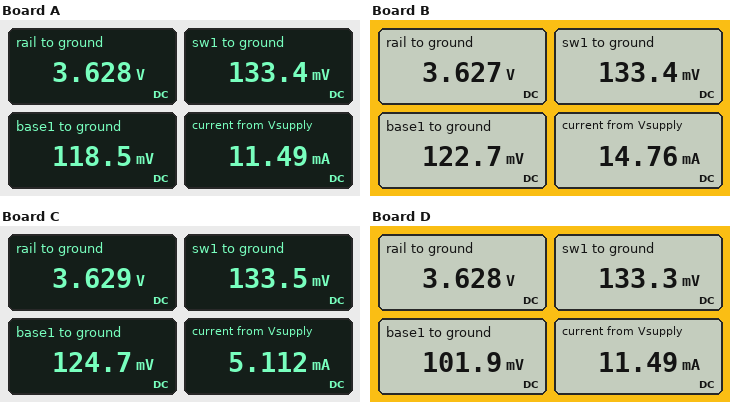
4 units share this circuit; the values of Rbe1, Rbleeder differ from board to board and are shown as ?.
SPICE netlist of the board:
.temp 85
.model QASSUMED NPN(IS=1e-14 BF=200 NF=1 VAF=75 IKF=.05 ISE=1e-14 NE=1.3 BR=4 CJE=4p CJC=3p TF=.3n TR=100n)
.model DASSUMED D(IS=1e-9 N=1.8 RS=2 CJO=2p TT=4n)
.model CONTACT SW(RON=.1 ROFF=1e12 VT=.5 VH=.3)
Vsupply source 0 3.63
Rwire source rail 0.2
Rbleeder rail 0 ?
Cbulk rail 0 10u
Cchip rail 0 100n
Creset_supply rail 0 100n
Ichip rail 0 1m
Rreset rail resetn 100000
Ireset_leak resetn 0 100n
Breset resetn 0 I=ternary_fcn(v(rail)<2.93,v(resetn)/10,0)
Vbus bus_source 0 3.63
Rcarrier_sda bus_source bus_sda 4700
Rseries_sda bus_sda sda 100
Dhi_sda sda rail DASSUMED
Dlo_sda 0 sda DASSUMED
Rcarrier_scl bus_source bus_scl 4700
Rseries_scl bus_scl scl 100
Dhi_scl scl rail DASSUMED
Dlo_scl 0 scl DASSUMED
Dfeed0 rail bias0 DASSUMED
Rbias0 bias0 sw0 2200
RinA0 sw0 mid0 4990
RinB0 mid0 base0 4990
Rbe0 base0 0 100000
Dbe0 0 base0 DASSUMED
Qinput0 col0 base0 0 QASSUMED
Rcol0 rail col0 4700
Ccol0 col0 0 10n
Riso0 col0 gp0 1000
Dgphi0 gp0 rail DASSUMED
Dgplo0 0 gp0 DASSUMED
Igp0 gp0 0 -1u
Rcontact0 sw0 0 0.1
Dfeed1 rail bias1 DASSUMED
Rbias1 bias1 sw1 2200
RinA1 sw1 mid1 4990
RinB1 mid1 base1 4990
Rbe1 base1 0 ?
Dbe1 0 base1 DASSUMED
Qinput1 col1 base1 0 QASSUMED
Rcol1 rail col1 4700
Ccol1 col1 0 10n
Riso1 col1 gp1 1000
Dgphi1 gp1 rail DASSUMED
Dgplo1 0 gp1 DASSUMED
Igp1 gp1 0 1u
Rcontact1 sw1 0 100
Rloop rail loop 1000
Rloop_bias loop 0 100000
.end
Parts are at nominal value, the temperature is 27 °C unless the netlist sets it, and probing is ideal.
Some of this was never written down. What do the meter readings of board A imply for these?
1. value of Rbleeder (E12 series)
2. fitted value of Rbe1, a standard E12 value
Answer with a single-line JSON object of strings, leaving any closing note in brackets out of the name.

{"value of Rbleeder": "470 Ω", "fitted value of Rbe1, a standard E12 value": "82 kΩ"}
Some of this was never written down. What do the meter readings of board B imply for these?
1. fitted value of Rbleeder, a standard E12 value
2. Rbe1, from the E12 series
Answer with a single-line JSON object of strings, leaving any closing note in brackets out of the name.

{"fitted value of Rbleeder, a standard E12 value": "330 Ω", "Rbe1, from the E12 series": "120 kΩ"}
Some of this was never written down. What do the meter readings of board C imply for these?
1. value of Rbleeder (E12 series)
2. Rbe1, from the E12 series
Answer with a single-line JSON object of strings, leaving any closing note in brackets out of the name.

{"value of Rbleeder": "2.7 kΩ", "Rbe1, from the E12 series": "150 kΩ"}
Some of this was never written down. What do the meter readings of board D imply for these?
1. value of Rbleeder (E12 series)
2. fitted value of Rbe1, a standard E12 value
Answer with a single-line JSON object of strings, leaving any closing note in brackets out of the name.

{"value of Rbleeder": "470 Ω", "fitted value of Rbe1, a standard E12 value": "33 kΩ"}
